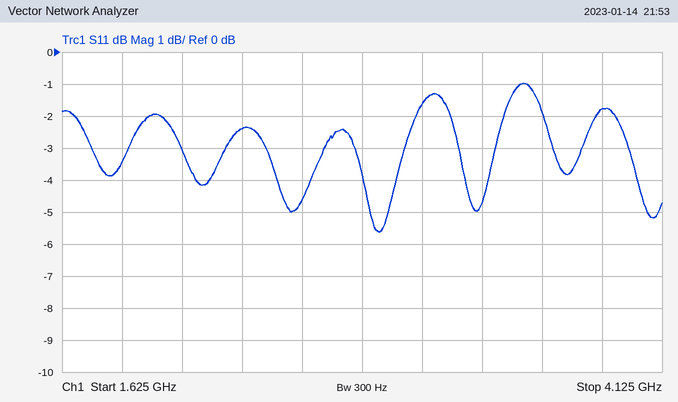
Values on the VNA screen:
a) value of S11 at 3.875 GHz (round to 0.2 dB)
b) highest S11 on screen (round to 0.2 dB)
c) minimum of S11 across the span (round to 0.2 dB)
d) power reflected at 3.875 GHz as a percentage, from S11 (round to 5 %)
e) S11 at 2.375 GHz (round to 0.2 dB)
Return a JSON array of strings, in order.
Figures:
["-1.8 dB", "-1.0 dB", "-5.6 dB", "65 %", "-2.4 dB"]
